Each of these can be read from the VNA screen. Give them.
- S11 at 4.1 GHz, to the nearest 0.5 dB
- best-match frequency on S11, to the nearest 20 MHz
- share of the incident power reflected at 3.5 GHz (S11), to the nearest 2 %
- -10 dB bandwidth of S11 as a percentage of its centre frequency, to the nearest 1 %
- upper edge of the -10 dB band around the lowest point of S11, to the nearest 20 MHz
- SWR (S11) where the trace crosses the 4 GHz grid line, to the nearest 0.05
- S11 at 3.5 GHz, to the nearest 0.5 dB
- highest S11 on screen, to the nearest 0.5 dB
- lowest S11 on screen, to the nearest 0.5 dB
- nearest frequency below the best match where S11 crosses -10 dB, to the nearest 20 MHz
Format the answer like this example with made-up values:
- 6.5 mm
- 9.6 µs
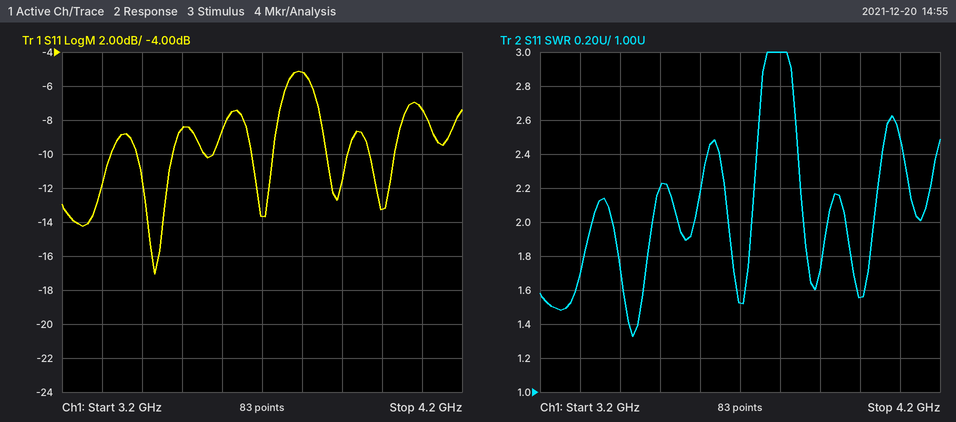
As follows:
- -7.5 dB
- 3.44 GHz
- 14 %
- 3 %
- 3.48 GHz
- 1.55
- -8.5 dB
- -5.0 dB
- -17.0 dB
- 3.38 GHz
